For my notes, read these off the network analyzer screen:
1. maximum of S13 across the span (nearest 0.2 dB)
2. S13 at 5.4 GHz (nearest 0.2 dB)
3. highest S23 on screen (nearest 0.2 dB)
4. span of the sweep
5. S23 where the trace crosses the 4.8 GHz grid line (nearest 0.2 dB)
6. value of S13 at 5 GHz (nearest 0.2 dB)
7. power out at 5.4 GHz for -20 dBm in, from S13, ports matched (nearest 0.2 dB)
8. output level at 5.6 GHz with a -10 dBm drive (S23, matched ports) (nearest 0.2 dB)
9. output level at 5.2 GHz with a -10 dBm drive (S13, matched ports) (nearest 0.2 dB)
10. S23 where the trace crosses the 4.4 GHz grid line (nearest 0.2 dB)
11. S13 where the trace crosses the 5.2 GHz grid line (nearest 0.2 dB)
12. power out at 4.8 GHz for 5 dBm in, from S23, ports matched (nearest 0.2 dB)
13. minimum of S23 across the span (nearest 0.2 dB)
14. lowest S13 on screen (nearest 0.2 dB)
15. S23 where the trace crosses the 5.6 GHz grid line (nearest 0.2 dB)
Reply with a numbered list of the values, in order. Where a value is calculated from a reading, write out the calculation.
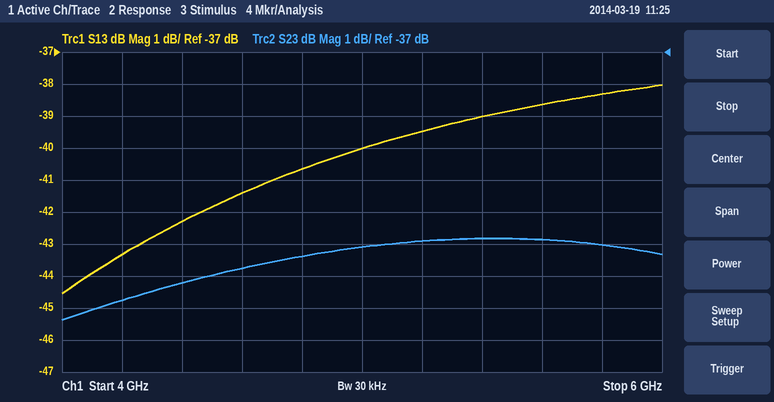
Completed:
1. -38.0 dB
2. -39.0 dB
3. -42.8 dB
4. 2 GHz
5. -43.4 dB
6. -40.0 dB
7. -20 dBm + (-39.0 dB) = -59.0 dBm
8. -10 dBm + (-42.8 dB) = -52.8 dBm
9. -10 dBm + (-39.4 dB) = -49.4 dBm
10. -44.2 dB
11. -39.4 dB
12. 5 dBm + (-43.4 dB) = -38.4 dBm
13. -45.4 dB
14. -44.6 dB
15. -42.8 dB
